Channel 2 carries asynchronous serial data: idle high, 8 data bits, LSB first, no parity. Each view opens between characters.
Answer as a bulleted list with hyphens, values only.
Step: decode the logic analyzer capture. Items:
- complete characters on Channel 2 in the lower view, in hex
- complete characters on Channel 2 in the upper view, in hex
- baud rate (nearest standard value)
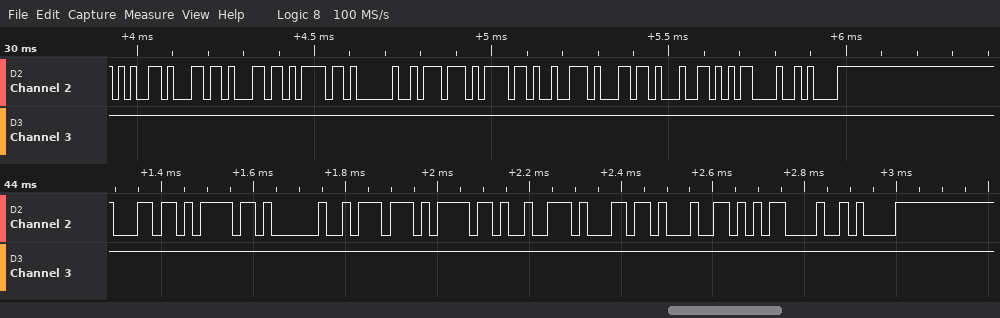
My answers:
- 6C, 6F, 20, 77, 6F, 72, 6C, 64, 0D, 0A
- 65, 6C, 6C, 6F, 20, 77, 6F, 72, 6C, 64, 0D, 0A
- 57600 baud
